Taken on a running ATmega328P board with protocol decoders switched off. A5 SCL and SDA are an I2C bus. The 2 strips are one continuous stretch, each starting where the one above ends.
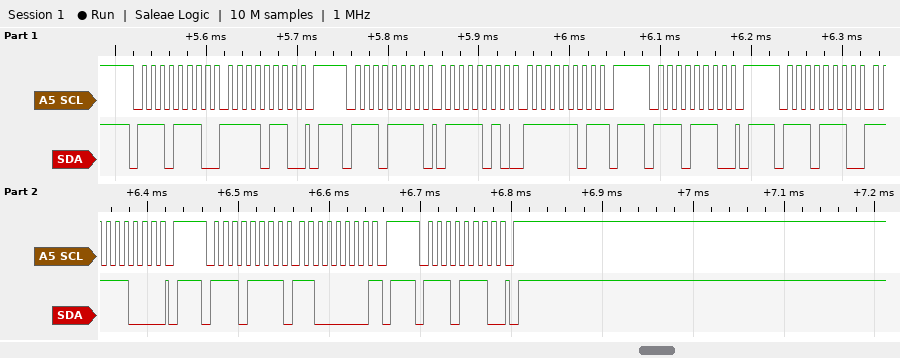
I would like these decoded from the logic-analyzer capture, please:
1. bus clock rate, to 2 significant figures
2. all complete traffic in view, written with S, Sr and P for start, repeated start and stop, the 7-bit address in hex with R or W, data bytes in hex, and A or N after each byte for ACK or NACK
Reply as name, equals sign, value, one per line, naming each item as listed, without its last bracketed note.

bus clock rate, to 2 significant figures = 100 kHz
all complete traffic in view, written with S, Sr and P for start, repeated start and stop, the 7-bit address in hex with R or W, data bytes in hex, and A or N after each byte for ACK or NACK = S 77W A F6 A P S 77R A 7A A FD N P S 77W A P S 77W A F8 A P S 77R A C0 N P S 77W A P
